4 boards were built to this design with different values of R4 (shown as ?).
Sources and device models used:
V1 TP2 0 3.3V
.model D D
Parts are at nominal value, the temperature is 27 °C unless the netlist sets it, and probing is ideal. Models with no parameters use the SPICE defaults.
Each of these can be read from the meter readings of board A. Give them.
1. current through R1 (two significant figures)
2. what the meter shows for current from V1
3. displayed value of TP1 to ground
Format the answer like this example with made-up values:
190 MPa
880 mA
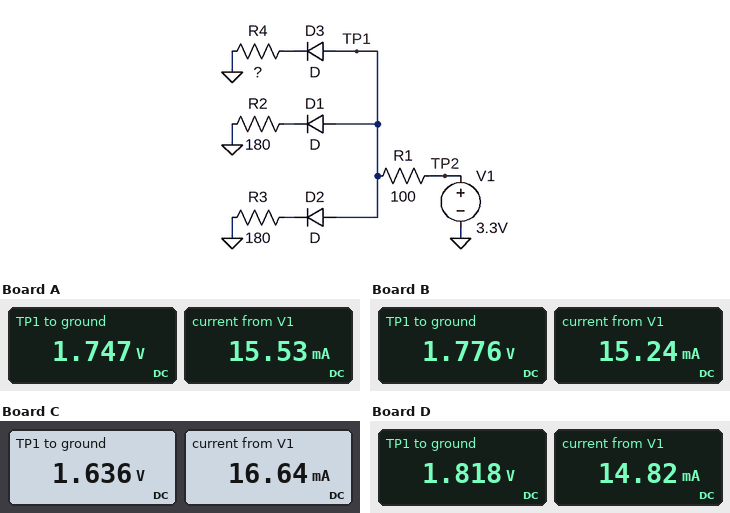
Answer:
16 mA
15.53 mA
1.747 V
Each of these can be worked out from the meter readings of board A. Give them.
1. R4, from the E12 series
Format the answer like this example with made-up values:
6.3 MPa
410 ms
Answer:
270 Ω
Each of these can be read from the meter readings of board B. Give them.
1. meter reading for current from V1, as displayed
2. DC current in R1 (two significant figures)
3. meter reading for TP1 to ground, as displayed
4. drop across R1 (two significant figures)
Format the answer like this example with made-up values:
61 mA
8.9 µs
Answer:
15.24 mA
15 mA
1.776 V
1.5 V
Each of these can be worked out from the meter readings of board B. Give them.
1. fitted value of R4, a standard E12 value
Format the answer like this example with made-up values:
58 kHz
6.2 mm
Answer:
330 Ω
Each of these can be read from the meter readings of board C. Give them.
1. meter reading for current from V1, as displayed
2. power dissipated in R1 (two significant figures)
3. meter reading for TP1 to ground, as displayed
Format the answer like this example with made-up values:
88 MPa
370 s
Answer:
16.64 mA
28 mW
1.636 V
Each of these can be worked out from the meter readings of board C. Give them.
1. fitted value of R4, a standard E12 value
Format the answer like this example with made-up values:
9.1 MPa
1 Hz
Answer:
150 Ω
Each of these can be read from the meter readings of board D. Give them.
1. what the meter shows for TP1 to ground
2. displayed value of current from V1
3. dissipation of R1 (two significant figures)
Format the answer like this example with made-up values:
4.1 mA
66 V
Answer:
1.818 V
14.82 mA
22 mW
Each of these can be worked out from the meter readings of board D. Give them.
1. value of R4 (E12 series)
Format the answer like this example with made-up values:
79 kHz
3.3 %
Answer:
470 Ω
